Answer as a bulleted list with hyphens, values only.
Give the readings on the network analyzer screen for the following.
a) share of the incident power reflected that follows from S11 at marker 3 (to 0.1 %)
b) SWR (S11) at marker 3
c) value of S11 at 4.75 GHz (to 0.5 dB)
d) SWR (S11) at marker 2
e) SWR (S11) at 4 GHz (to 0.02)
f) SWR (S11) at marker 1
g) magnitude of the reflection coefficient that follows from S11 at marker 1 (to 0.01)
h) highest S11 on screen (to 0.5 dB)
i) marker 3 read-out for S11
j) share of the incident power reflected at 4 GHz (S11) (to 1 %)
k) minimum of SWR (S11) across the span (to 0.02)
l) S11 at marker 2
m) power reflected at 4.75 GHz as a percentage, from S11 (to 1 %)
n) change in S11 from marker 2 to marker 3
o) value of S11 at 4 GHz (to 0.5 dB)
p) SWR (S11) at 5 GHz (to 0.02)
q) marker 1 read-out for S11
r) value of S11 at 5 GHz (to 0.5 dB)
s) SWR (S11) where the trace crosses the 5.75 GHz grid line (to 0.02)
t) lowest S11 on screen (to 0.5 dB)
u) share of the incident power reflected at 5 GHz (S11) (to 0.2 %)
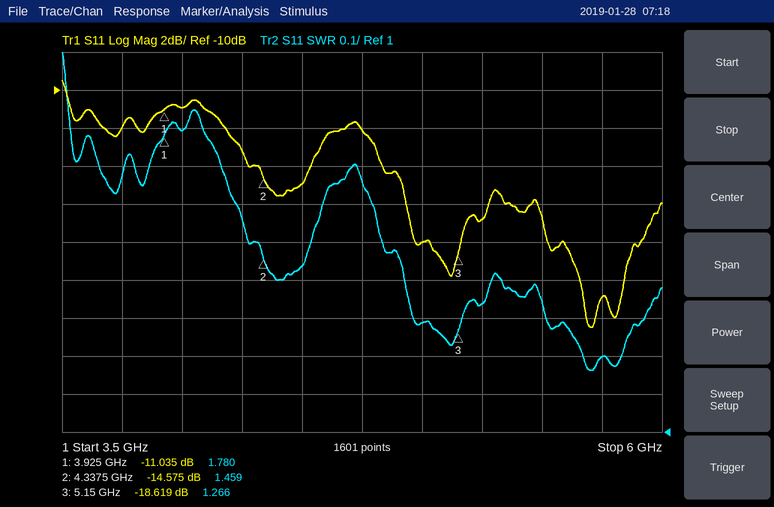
- 1.4 %
- 1.266
- -12.0 dB
- 1.459
- 1.80
- 1.780
- 0.28
- -9.5 dB
- -18.619 dB
- 8 %
- 1.16
- -14.575 dB
- 6 %
- -4.044 dB
- -11.0 dB
- 1.28
- -11.035 dB
- -18.0 dB
- 1.20
- -22.5 dB
- 1.6 %
